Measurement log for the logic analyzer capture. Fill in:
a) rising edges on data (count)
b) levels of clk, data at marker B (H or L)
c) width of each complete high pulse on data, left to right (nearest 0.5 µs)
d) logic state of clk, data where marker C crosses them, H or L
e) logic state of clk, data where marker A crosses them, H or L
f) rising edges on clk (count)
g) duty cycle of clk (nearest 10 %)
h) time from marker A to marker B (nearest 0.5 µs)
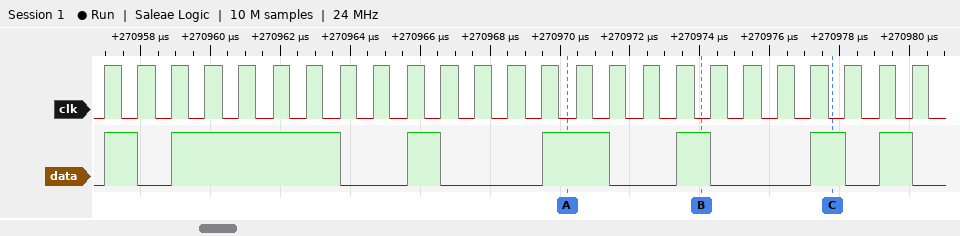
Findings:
7
clk=L, data=H
1 µs, 5 µs, 1 µs, 2 µs, 1 µs, 1 µs, 1 µs
clk=L, data=H
clk=L, data=H
25
50 %
4 µs
